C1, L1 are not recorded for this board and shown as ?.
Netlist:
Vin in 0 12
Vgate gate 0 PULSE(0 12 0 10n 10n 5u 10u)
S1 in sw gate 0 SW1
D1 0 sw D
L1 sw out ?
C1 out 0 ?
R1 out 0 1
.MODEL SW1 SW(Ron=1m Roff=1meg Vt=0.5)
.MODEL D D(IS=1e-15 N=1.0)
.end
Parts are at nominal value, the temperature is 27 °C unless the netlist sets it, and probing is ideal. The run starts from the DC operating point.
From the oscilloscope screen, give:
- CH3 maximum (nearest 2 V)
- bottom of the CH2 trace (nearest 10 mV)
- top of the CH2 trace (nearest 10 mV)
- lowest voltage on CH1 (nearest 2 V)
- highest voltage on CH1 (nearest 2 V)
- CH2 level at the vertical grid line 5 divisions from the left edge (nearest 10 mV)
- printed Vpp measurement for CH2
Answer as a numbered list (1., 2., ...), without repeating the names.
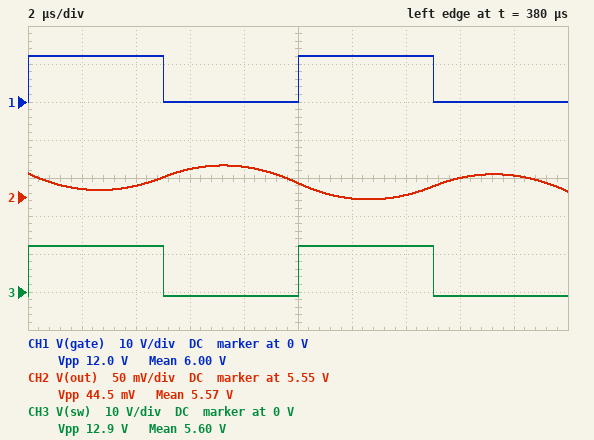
1. 12 V
2. 5.55 V
3. 5.59 V
4. 0 V
5. 12 V
6. 5.57 V
7. 44.5 mV
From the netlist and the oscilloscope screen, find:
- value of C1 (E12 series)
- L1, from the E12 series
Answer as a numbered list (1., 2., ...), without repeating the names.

1. 39 µF
2. 27 µH
